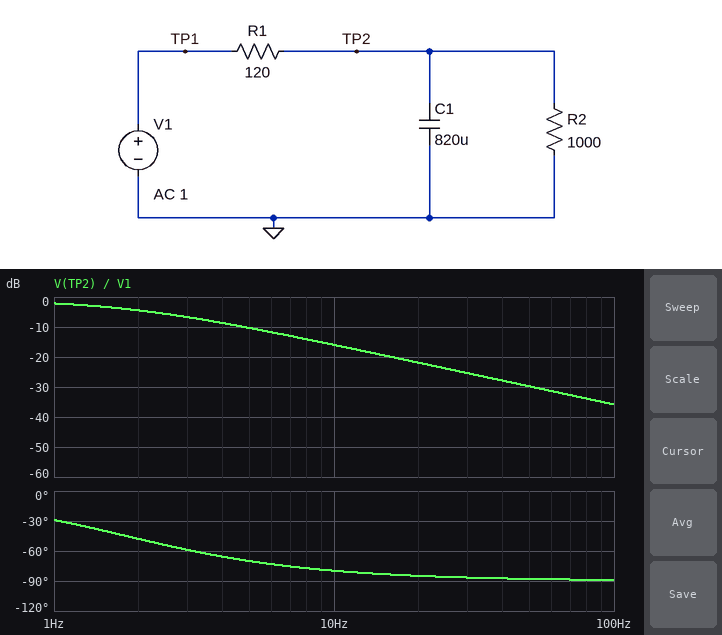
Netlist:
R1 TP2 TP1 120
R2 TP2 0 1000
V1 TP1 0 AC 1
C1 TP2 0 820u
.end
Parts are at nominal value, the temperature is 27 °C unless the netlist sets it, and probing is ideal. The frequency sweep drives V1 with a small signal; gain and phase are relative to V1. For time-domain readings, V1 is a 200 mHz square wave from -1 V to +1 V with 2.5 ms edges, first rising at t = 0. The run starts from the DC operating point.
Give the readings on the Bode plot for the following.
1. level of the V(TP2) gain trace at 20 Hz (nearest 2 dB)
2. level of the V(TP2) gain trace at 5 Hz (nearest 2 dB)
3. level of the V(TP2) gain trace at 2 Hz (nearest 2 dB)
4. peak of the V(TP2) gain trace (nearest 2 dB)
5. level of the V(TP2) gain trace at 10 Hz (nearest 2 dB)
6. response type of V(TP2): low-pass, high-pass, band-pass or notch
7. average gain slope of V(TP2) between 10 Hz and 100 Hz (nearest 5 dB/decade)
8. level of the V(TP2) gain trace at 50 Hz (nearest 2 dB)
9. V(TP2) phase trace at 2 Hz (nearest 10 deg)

-22 dB
-10 dB
-4 dB
-2 dB
-16 dB
low-pass
-20 dB/decade
-30 dB
-50 deg
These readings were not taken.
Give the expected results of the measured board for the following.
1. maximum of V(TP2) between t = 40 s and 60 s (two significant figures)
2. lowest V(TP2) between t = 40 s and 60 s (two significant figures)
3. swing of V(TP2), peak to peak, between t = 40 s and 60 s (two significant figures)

890 mV
-890 mV
1.8 V
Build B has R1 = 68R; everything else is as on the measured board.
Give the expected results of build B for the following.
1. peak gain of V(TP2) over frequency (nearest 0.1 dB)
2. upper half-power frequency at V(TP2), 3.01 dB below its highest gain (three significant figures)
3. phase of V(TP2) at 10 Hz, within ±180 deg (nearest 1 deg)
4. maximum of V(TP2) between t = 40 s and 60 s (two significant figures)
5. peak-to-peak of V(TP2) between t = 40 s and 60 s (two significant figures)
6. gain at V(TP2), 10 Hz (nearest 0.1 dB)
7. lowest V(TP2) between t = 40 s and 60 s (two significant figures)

-0.6 dB
3.05 Hz
-73 deg
940 mV
1.9 V
-11.3 dB
-940 mV
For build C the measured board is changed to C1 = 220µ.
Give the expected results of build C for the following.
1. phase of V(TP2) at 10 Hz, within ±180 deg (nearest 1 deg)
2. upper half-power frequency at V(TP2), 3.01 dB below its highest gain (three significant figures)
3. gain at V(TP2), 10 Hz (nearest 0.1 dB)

-56 deg
6.75 Hz
-6.0 dB
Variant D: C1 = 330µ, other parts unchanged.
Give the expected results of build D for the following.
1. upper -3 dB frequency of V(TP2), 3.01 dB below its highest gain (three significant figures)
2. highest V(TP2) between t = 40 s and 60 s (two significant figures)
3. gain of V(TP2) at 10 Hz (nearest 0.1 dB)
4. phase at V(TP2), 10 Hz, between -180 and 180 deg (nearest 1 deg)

4.50 Hz
890 mV
-8.7 dB
-66 deg
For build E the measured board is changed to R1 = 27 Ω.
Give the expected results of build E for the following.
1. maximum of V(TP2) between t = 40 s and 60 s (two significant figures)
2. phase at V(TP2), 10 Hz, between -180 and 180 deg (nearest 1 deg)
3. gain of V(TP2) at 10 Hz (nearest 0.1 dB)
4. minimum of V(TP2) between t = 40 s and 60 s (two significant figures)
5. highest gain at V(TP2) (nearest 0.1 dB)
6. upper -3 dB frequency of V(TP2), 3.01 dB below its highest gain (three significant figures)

970 mV
-54 deg
-4.8 dB
-970 mV
-0.2 dB
7.38 Hz
